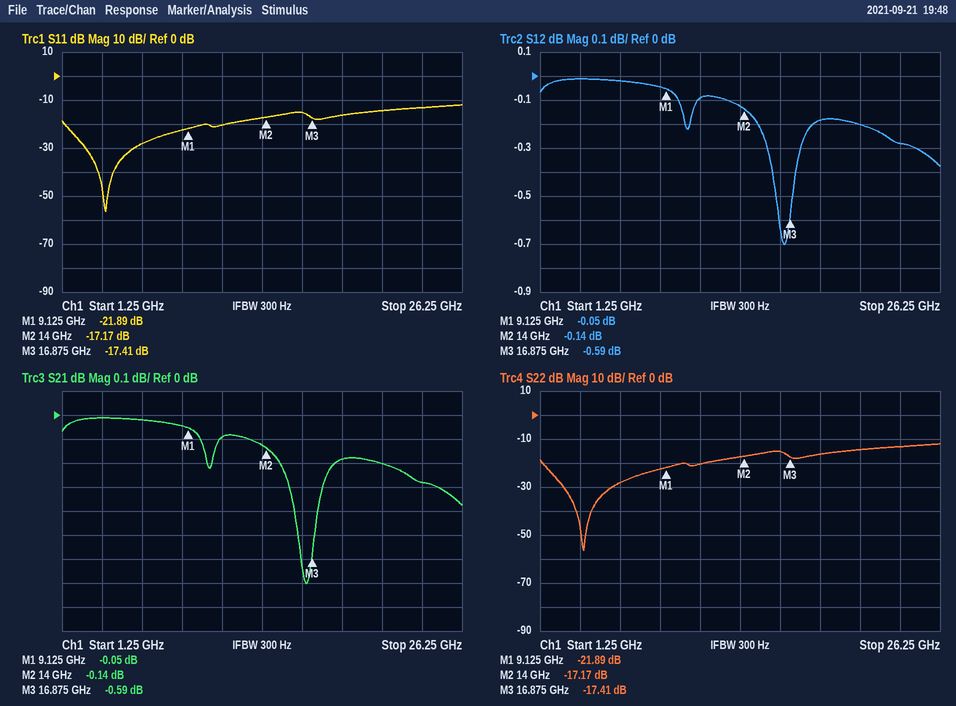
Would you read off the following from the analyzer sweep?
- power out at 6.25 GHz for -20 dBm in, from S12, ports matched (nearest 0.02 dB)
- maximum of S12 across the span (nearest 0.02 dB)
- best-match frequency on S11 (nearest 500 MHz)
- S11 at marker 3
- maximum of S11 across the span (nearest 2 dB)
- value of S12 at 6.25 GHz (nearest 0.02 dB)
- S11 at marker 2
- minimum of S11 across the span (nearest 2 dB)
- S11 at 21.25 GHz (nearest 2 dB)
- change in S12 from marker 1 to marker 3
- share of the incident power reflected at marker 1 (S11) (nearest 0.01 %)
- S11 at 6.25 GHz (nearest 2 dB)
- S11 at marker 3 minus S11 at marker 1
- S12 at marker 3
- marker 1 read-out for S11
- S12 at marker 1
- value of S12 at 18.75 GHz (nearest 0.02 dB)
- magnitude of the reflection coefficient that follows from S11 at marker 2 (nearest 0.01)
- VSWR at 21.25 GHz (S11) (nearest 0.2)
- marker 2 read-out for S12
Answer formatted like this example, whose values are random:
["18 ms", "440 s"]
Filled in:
["-20.02 dBm", "-0.02 dB", "4.0 GHz", "-17.41 dB", "-12 dB", "-0.02 dB", "-17.17 dB", "-56 dB", "-14 dB", "-0.54 dB", "0.65 %", "-28 dB", "4.48 dB", "-0.59 dB", "-21.89 dB", "-0.05 dB", "-0.18 dB", "0.14", "1.4", "-0.14 dB"]
